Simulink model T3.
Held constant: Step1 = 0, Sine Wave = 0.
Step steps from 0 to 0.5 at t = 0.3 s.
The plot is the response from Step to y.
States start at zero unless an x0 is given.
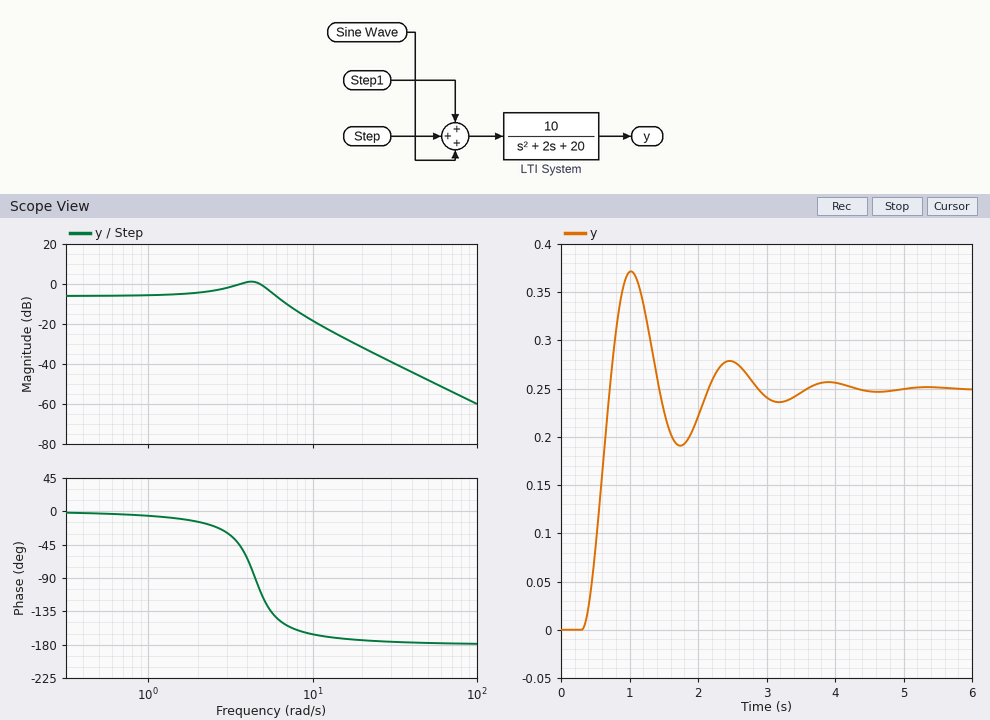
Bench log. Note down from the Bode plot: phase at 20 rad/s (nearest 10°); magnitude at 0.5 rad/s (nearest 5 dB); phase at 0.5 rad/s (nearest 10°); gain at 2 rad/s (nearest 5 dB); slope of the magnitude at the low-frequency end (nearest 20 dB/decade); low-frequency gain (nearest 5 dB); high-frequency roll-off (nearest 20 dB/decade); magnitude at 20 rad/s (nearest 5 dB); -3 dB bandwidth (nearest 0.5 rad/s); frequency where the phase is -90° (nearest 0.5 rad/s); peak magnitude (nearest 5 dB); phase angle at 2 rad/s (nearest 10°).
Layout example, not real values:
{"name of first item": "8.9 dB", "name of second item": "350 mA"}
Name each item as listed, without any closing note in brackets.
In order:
{"phase at 20 rad/s": "-170°", "magnitude at 0.5 rad/s": "-5 dB", "phase at 0.5 rad/s": "0°", "gain at 2 rad/s": "-5 dB", "slope of the magnitude at the low-frequency end": "0 dB/decade", "low-frequency gain": "-5 dB", "high-frequency roll-off": "-40 dB/decade", "magnitude at 20 rad/s": "-30 dB", "-3 dB bandwidth": "6.5 rad/s", "frequency where the phase is -90°": "4.5 rad/s", "peak magnitude": "0 dB", "phase angle at 2 rad/s": "-10°"}
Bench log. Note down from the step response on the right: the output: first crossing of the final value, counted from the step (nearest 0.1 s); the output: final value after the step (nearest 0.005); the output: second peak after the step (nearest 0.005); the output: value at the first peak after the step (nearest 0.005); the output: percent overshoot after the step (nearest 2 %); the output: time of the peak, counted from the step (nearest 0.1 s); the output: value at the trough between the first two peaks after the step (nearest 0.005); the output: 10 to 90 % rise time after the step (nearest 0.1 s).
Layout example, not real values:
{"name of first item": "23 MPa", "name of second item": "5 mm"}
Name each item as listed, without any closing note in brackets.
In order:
{"the output: first crossing of the final value, counted from the step": "0.4 s", "the output: final value after the step": "0.250", "the output: second peak after the step": "0.280", "the output: value at the first peak after the step": "0.370", "the output: percent overshoot after the step": "48 %", "the output: time of the peak, counted from the step": "0.7 s", "the output: value at the trough between the first two peaks after the step": "0.190", "the output: 10 to 90 % rise time after the step": "0.3 s"}
